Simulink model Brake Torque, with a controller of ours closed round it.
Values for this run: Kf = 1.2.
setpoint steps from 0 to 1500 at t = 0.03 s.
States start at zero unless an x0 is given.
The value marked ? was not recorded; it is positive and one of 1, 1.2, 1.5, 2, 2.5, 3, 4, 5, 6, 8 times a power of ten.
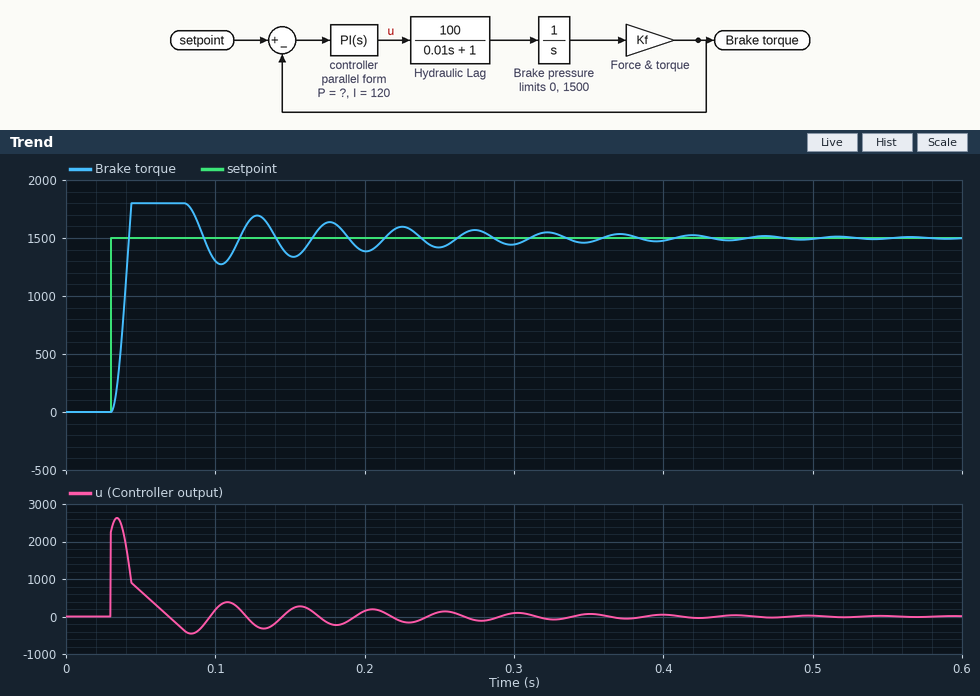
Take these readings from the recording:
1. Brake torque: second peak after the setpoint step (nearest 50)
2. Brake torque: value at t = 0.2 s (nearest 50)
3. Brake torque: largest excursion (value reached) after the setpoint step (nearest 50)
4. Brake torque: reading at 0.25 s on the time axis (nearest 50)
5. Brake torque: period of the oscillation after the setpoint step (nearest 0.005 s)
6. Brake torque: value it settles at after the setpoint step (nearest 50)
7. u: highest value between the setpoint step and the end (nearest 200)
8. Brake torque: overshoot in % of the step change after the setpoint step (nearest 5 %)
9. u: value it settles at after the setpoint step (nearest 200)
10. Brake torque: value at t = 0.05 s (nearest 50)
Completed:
1700
1400
1800
1400
0.065 s
1500
2600
20 %
0
1800
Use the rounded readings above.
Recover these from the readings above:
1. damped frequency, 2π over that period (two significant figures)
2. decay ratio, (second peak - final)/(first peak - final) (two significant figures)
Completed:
97 rad/s
0.67
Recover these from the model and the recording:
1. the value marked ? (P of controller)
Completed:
1.5
